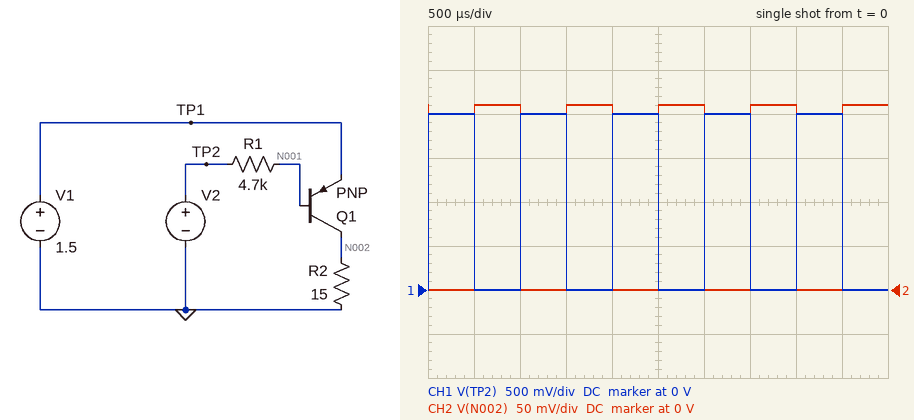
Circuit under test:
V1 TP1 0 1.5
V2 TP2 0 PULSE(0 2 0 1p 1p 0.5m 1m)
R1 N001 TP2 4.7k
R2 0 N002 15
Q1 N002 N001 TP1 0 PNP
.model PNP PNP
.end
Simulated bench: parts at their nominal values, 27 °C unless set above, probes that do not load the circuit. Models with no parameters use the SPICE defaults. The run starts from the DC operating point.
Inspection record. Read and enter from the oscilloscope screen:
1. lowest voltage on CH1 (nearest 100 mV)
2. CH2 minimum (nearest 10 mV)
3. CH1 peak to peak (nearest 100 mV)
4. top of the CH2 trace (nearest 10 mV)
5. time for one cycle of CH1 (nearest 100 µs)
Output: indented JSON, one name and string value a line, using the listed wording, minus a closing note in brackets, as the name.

{
  "lowest voltage on CH1": "0 V",
  "CH2 minimum": "0 V",
  "CH1 peak to peak": "2.0 V",
  "top of the CH2 trace": "210 mV",
  "time for one cycle of CH1": "1.0 ms"
}
